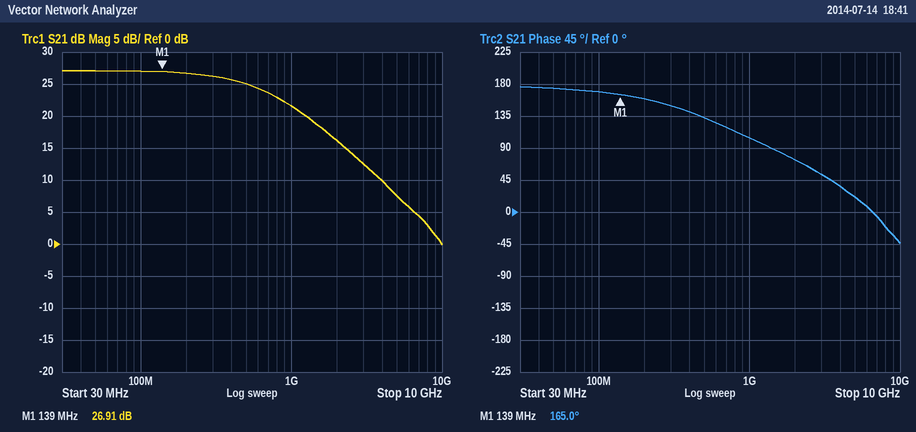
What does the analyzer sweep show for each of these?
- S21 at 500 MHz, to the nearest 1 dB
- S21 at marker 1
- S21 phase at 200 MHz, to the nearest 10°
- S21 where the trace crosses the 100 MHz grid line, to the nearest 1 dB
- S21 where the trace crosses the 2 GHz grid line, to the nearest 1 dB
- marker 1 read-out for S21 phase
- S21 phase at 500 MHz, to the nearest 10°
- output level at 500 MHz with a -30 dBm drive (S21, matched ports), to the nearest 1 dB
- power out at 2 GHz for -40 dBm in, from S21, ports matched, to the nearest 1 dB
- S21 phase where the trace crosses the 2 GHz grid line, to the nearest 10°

25 dB
26.91 dB
160°
27 dB
16 dB
165.0°
130°
-5 dBm
-24 dBm
70°
